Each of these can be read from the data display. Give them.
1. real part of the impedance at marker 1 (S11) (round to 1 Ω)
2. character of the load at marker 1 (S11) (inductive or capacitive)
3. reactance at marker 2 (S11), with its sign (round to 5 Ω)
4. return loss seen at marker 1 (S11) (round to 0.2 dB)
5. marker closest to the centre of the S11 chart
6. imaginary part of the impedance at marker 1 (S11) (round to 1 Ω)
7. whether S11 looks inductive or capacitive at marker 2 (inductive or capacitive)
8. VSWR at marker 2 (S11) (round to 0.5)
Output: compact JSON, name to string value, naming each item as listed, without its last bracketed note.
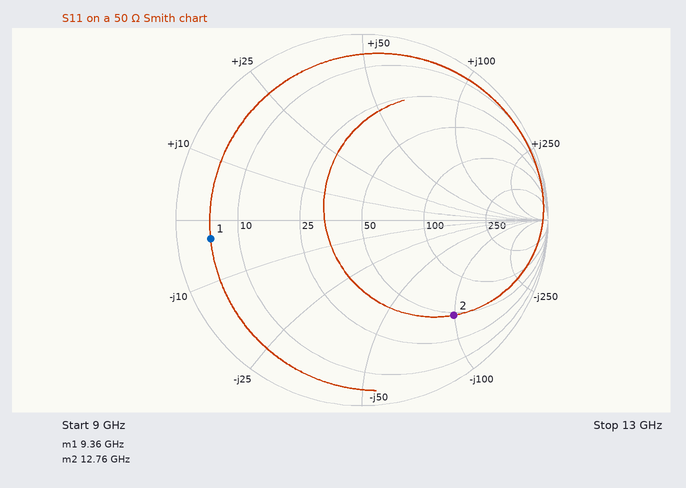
{"real part of the impedance at marker 1 (S11)": "5 Ω", "character of the load at marker 1 (S11)": "capacitive", "reactance at marker 2 (S11), with its sign": "-100 Ω", "return loss seen at marker 1 (S11)": "1.8 dB", "marker closest to the centre of the S11 chart": "marker 2", "imaginary part of the impedance at marker 1 (S11)": "-3 Ω", "whether S11 looks inductive or capacitive at marker 2": "capacitive", "VSWR at marker 2 (S11)": "6.0"}
